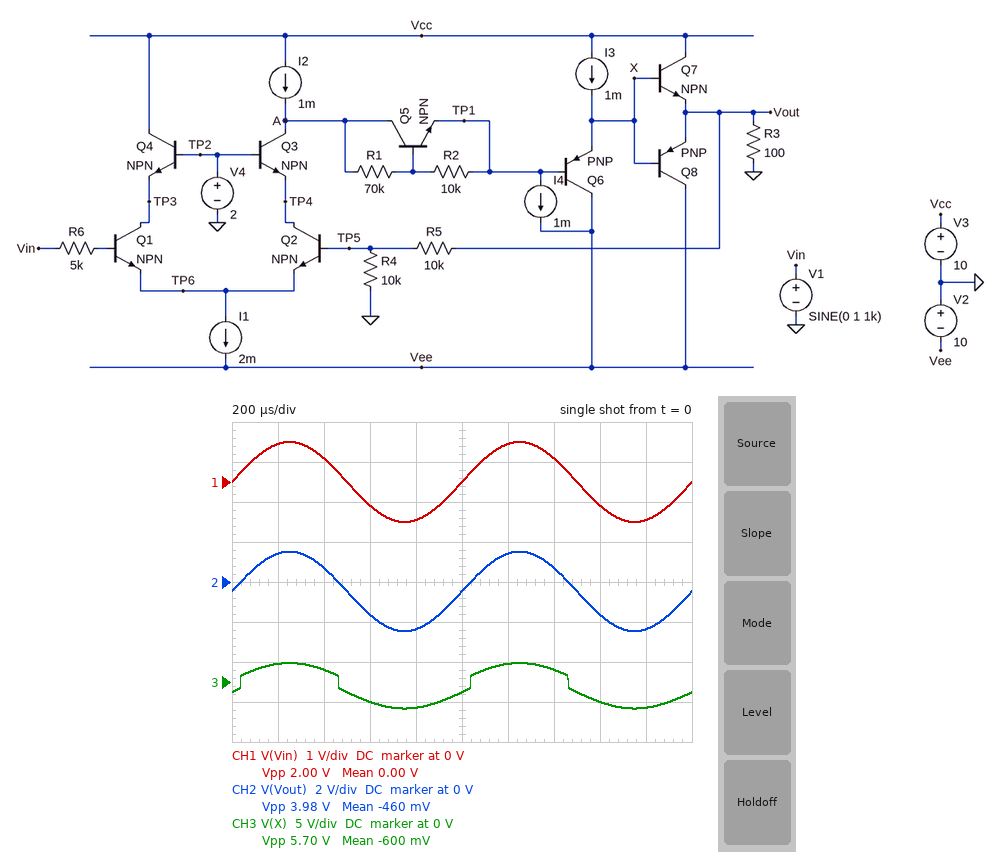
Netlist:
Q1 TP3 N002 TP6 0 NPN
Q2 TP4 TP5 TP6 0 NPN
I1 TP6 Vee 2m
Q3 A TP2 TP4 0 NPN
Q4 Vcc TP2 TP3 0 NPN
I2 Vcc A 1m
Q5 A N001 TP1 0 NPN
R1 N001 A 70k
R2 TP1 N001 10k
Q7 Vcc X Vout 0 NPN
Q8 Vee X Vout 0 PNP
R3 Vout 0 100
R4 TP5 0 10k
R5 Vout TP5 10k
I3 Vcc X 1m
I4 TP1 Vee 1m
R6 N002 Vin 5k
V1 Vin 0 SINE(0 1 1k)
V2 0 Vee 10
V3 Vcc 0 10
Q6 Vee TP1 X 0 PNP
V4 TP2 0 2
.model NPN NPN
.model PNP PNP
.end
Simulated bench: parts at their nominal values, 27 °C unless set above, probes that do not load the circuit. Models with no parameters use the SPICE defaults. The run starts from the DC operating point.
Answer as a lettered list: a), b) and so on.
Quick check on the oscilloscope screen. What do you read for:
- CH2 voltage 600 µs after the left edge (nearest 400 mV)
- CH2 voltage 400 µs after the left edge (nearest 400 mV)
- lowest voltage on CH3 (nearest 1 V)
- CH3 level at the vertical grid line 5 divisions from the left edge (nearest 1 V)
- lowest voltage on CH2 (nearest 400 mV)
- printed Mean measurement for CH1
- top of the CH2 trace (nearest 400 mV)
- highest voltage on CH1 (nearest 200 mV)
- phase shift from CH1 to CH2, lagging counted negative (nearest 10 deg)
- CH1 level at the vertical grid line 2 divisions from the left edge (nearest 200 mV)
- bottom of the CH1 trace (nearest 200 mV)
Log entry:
a) -1.6 V
b) 800 mV
c) -3 V
d) -1 V
e) -2.4 V
f) 0.00 V
g) 1.6 V
h) 1.0 V
i) 0 deg
j) 600 mV
k) -1.0 V
